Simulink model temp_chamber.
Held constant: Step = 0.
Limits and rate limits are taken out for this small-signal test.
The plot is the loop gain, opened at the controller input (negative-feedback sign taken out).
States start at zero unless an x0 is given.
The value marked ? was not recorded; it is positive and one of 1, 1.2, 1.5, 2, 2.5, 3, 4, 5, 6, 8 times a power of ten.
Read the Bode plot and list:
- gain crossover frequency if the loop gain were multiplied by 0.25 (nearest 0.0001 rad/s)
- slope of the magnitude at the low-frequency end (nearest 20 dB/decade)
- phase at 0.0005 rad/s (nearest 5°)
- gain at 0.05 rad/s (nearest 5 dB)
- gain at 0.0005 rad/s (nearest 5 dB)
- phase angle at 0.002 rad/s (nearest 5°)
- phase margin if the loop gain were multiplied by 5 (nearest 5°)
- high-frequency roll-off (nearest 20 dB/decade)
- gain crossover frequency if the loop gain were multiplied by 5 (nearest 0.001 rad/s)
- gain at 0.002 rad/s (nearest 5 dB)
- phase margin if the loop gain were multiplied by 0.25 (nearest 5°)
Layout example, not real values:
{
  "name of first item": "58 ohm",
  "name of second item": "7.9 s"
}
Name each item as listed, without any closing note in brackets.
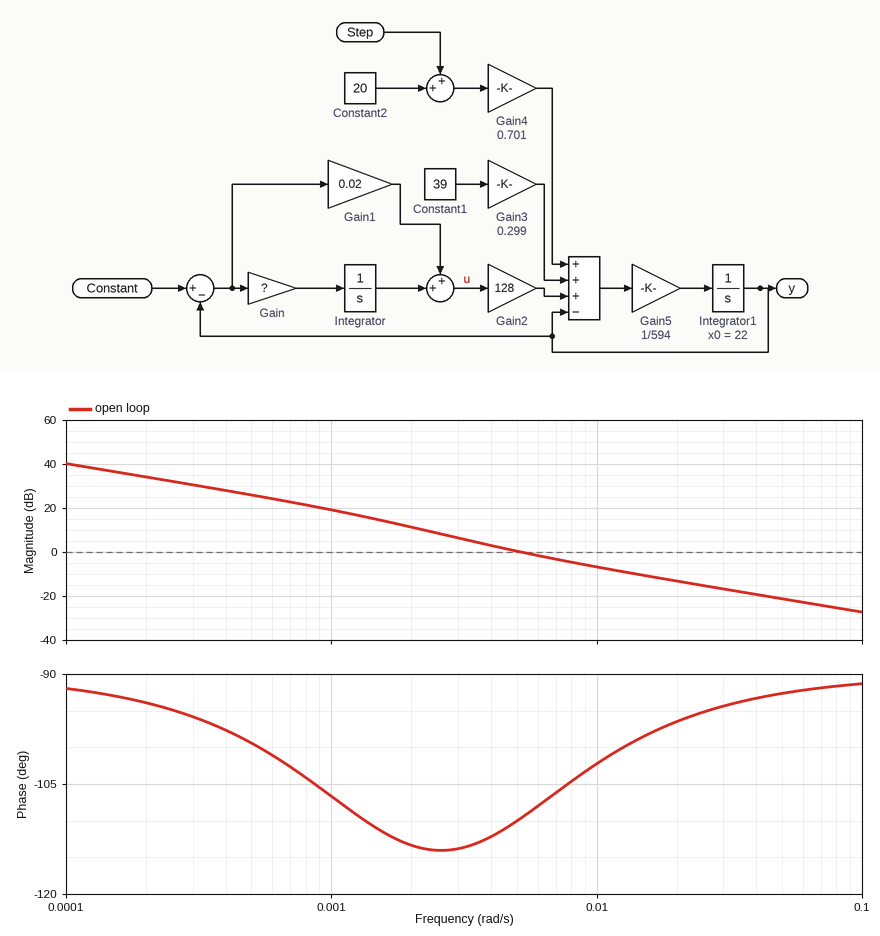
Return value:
{
  "gain crossover frequency if the loop gain were multiplied by 0.25": "0.0019 rad/s",
  "slope of the magnitude at the low-frequency end": "-20 dB/decade",
  "phase at 0.0005 rad/s": "-100°",
  "gain at 0.05 rad/s": "-20 dB",
  "gain at 0.0005 rad/s": "25 dB",
  "phase angle at 0.002 rad/s": "-115°",
  "phase margin if the loop gain were multiplied by 5": "85°",
  "high-frequency roll-off": "-20 dB/decade",
  "gain crossover frequency if the loop gain were multiplied by 5": "0.022 rad/s",
  "gain at 0.002 rad/s": "10 dB",
  "phase margin if the loop gain were multiplied by 0.25": "65°"
}
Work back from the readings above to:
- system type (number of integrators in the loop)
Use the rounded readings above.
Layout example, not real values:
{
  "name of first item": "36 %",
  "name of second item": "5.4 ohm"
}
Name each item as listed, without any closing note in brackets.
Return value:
{
  "system type": "1"
}
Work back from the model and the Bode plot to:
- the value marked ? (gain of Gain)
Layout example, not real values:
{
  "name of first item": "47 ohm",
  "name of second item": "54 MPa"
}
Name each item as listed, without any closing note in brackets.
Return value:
{
  "the value marked ?": "8e-05"
}
